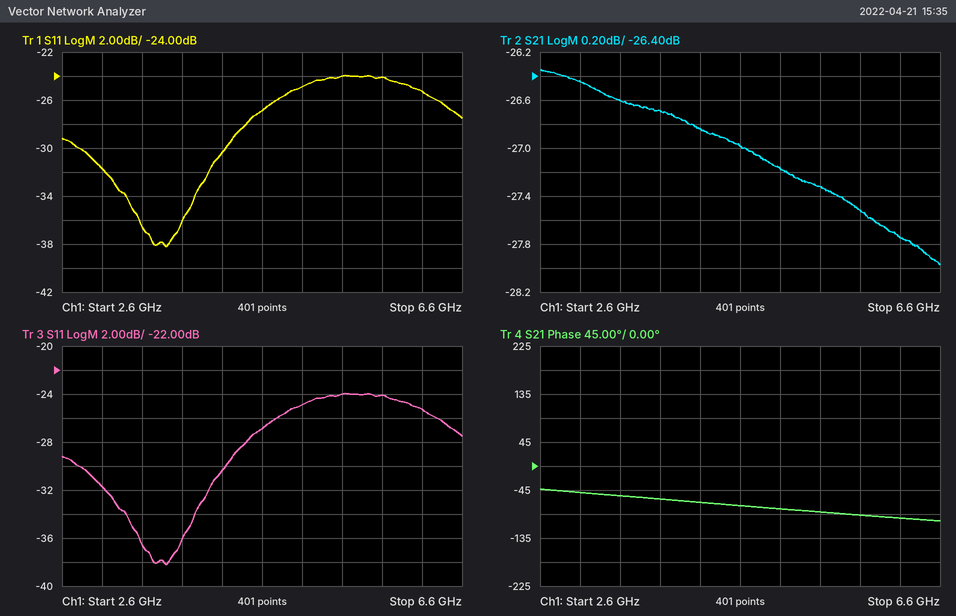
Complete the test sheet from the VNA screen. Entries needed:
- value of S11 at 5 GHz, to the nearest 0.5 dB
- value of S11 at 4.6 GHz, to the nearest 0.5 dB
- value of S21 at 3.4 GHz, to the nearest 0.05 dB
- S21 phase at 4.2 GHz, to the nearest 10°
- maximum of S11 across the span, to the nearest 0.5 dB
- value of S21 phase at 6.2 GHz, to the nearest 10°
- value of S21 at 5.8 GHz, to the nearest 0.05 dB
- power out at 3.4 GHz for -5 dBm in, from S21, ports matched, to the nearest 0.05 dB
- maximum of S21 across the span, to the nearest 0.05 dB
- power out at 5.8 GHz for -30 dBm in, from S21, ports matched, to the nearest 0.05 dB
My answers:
-25.0 dB
-27.0 dB
-26.60 dB
-70°
-24.0 dB
-100°
-27.50 dB
-31.60 dBm
-26.35 dB
-57.50 dBm
